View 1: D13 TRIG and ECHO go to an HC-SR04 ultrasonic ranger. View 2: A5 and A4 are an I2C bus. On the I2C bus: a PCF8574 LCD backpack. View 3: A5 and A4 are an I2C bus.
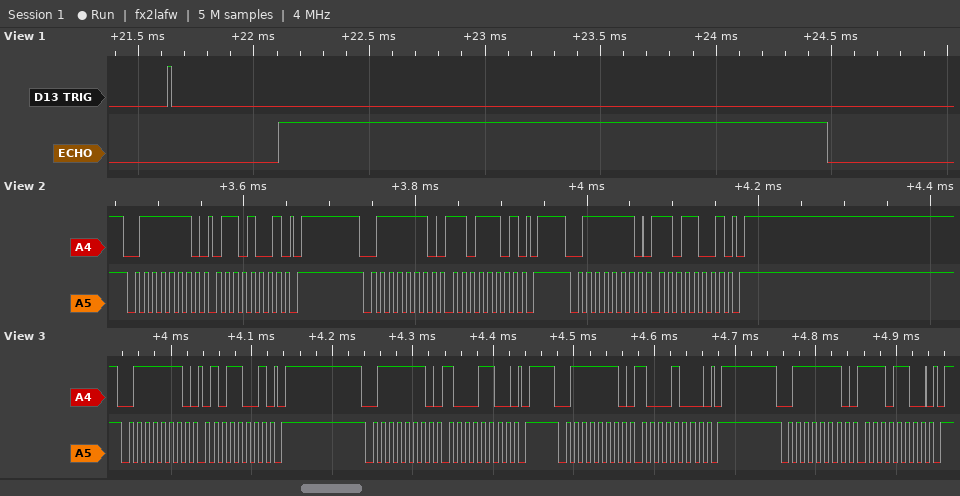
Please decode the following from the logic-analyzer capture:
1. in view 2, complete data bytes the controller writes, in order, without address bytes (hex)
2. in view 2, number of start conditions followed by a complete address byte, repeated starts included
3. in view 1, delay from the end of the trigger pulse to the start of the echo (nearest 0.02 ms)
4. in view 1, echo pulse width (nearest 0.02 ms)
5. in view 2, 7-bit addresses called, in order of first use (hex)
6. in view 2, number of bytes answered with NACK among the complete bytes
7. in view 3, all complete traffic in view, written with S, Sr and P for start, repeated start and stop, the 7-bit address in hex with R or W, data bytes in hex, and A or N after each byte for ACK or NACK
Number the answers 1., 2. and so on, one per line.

1. 69 DD D9
2. 3
3. 0.46 ms
4. 2.38 ms
5. 0x3F
6. 0
7. S 3FW A 59 A P S 3FW A 8C A P S 3FW A 88 A P S 3FW A EC A P
